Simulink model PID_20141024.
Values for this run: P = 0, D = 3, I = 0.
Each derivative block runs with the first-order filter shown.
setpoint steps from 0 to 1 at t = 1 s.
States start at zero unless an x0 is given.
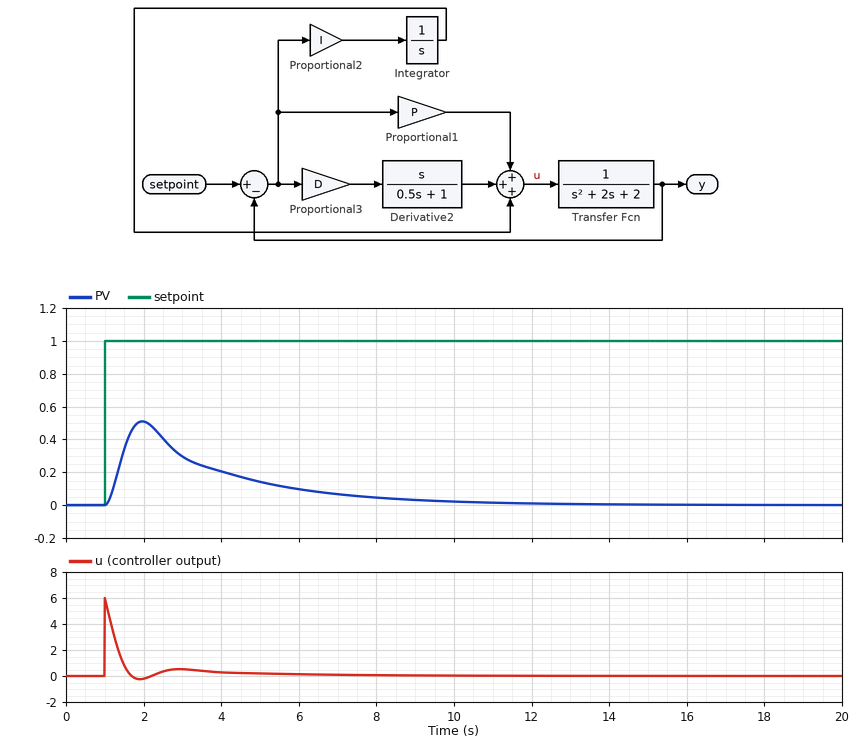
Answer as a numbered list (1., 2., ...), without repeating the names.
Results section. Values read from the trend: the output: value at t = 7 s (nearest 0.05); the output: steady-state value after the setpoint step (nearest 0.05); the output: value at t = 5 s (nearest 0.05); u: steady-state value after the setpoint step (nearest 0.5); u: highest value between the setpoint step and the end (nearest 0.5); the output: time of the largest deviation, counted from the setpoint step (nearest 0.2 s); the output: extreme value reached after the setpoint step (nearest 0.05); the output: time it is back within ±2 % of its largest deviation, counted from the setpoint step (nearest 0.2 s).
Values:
1. 0.05
2. 0.00
3. 0.15
4. 0.0
5. 6.0
6. 1.0 s
7. 0.50
8. 11.0 s
